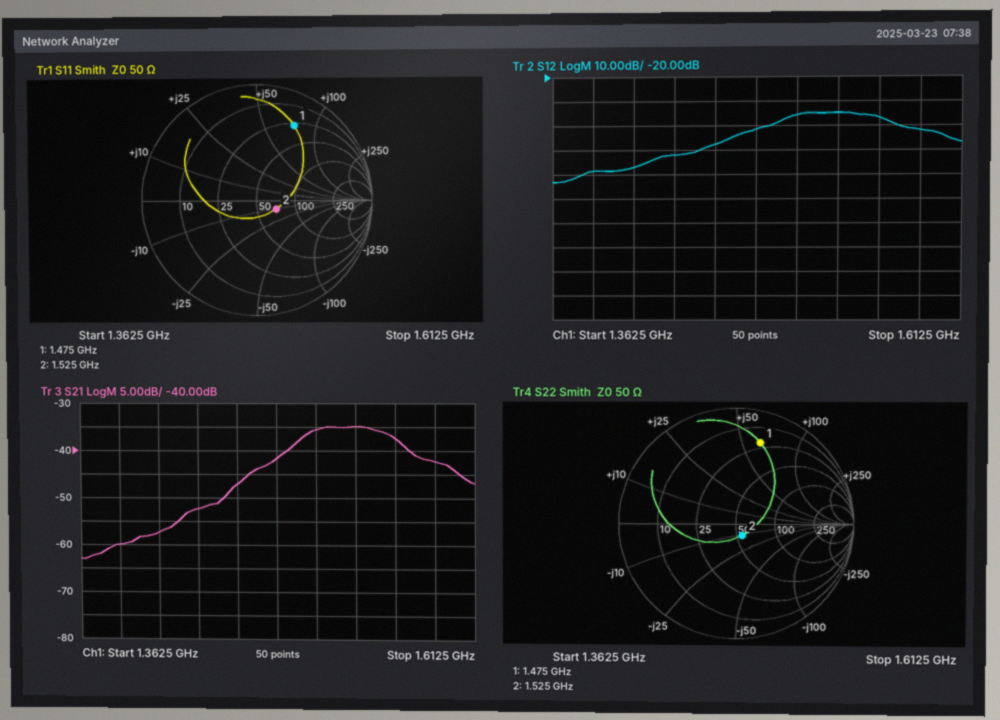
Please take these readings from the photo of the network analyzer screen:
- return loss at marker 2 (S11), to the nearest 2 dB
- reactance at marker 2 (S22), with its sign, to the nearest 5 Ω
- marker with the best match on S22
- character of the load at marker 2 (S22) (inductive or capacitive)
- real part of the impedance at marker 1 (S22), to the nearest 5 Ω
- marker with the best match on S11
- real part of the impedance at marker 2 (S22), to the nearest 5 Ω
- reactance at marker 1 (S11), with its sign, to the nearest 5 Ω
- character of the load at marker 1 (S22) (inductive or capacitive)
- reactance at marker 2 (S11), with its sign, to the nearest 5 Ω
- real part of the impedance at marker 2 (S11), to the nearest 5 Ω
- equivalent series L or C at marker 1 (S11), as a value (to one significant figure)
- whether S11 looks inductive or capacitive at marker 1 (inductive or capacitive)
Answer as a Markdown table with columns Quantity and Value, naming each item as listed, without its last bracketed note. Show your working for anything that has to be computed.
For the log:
| Quantity | Value |
|---|---|
| return loss at marker 2 (S11), to the nearest 2 dB | 14 dB |
| reactance at marker 2 (S22), with its sign, to the nearest 5 Ω | -10 Ω |
| marker with the best match on S22 | marker 2 |
| character of the load at marker 2 (S22) | capacitive |
| real part of the impedance at marker 1 (S22), to the nearest 5 Ω | 20 Ω |
| marker with the best match on S11 | marker 2 |
| real part of the impedance at marker 2 (S22), to the nearest 5 Ω | 55 Ω |
| reactance at marker 1 (S11), with its sign, to the nearest 5 Ω | +75 Ω |
| character of the load at marker 1 (S22) | inductive |
| reactance at marker 2 (S11), with its sign, to the nearest 5 Ω | -10 Ω |
| real part of the impedance at marker 2 (S11), to the nearest 5 Ω | 70 Ω |
| equivalent series L or C at marker 1 (S11), as a value | L = 75 Ω/(2π × 1.475 GHz) ≈ 8 nH |
| whether S11 looks inductive or capacitive at marker 1 | inductive |
